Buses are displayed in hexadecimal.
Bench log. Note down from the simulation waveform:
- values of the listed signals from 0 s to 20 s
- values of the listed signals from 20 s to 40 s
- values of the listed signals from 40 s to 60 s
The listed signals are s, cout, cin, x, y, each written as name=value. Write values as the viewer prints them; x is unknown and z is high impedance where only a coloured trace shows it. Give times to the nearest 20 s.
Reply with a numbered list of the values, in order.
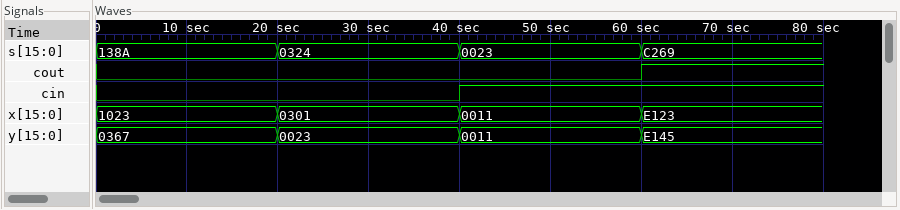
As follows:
1. s=138A, cout=0, cin=0, x=1023, y=0367
2. s=0324, cout=0, cin=0, x=0301, y=0023
3. s=0023, cout=0, cin=1, x=0011, y=0011
